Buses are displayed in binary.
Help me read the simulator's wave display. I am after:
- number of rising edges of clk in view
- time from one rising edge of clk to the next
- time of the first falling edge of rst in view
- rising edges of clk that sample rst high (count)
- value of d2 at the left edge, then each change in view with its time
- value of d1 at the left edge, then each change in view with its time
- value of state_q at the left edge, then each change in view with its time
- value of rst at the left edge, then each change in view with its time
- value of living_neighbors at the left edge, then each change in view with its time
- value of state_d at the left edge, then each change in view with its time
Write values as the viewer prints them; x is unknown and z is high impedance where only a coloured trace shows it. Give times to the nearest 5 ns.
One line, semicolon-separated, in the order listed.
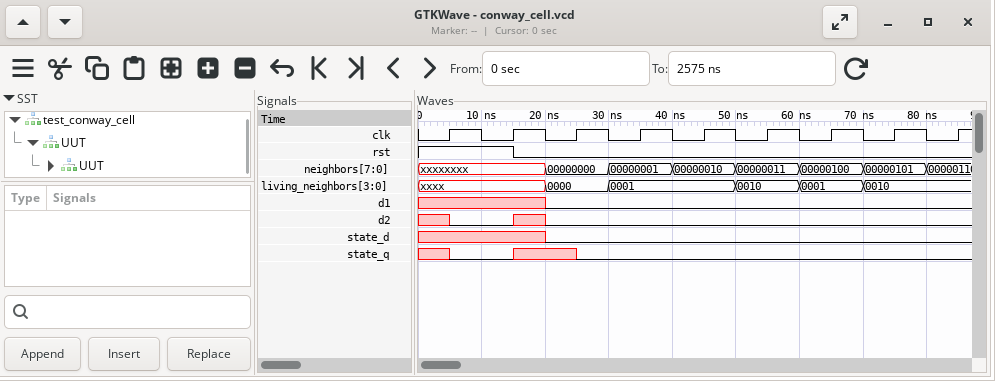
9; 10 ns; 15 ns; 2; x, 0 at 5 ns, x at 15 ns, 0 at 20 ns; x, 0 at 20 ns; x, 0 at 5 ns, x at 15 ns, 0 at 25 ns; 1, 0 at 15 ns; xxxx, 0000 at 20 ns, 0001 at 30 ns, 0010 at 50 ns, 0001 at 60 ns, 0010 at 70 ns; x, 0 at 20 ns
